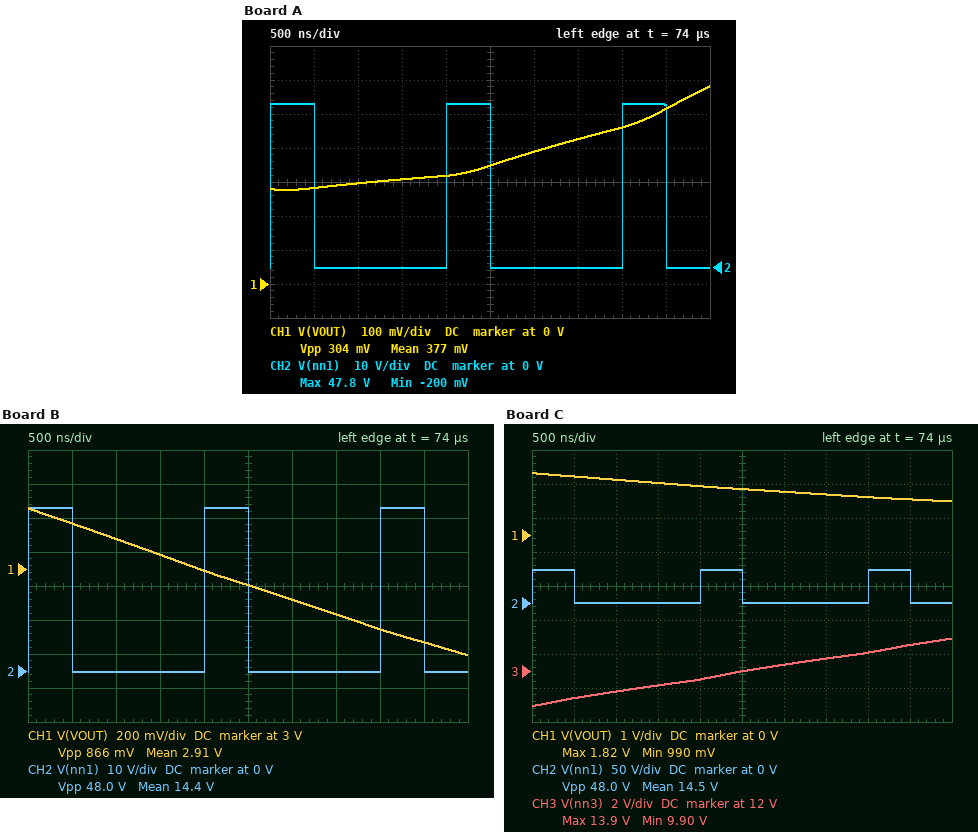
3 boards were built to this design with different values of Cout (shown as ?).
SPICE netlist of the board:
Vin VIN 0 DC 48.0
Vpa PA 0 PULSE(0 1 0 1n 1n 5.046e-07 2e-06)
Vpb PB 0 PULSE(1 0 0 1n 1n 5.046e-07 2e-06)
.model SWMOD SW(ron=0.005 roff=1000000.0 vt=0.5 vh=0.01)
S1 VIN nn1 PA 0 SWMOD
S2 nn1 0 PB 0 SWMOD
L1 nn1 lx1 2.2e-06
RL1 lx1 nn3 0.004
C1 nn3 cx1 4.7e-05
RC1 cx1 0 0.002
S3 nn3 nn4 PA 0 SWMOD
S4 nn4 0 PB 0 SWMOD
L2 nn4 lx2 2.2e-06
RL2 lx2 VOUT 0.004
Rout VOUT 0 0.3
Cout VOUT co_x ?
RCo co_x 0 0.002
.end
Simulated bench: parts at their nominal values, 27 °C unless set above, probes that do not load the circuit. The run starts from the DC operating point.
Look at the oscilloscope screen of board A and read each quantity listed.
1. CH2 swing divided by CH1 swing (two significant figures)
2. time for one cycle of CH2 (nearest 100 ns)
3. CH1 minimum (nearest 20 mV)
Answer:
160
2.0 µs
280 mV
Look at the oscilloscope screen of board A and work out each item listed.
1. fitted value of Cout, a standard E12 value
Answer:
33 µF
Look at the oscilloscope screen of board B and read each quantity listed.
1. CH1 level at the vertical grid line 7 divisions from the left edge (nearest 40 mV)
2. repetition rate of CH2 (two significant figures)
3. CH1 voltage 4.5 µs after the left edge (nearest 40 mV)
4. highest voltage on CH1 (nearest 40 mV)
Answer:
2.72 V
500 kHz
2.56 V
3.36 V
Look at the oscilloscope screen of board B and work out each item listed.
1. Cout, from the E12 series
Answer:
120 µF
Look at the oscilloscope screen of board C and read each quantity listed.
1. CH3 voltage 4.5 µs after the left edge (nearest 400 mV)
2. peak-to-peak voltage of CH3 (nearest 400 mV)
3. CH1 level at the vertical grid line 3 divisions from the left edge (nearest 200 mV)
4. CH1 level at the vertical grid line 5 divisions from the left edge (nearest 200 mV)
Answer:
13.6 V
4.0 V
1.6 V
1.4 V
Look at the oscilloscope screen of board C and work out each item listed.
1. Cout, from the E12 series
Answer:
82 µF
